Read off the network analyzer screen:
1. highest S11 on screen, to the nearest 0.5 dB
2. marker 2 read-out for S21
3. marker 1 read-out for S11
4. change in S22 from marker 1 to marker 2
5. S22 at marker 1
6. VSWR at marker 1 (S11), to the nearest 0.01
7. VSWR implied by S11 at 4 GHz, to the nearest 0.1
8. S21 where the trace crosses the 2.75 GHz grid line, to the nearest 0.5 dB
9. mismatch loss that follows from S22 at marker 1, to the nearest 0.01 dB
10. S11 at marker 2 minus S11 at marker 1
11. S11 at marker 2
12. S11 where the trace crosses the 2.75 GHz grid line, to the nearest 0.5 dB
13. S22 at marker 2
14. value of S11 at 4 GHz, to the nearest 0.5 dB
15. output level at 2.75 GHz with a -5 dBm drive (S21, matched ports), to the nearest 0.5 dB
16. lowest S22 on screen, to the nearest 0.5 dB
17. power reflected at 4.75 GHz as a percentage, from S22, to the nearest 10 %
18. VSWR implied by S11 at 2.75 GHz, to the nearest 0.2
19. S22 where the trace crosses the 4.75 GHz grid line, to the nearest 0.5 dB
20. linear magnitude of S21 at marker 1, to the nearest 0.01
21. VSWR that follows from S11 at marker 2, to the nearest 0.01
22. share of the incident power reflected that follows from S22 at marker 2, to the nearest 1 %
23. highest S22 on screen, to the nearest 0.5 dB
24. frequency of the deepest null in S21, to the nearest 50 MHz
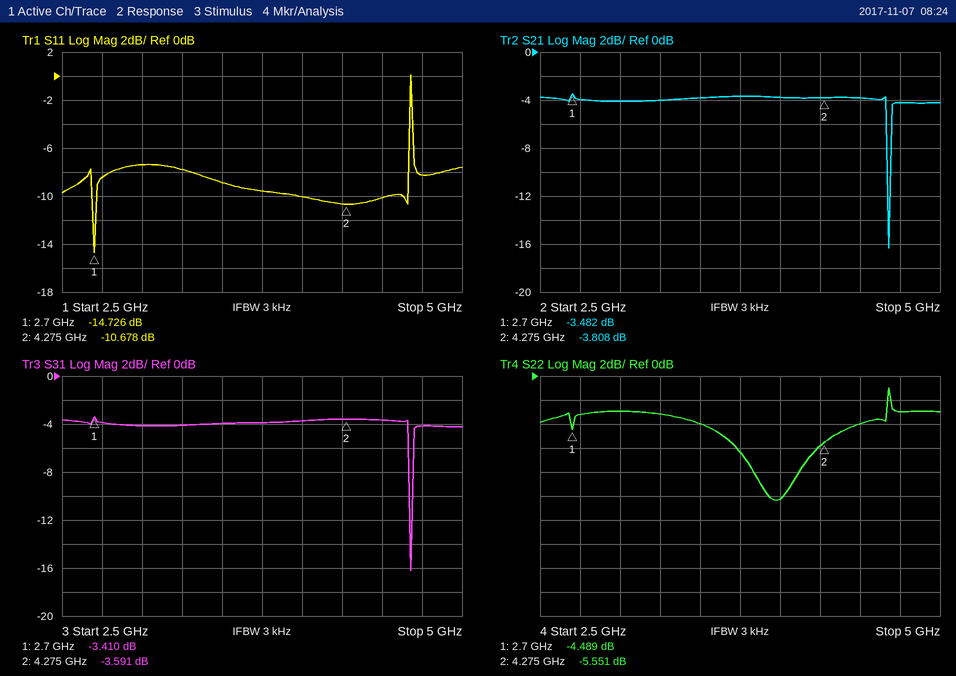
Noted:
0.0 dB
-3.808 dB
-14.726 dB
-1.062 dB
-4.489 dB
1.45
1.9
-4.0 dB
1.91 dB
4.048 dB
-10.678 dB
-8.5 dB
-5.551 dB
-10.0 dB
-9.0 dBm
-10.5 dB
50 %
2.2
-3.0 dB
0.67
1.83
28 %
-1.0 dB
4.70 GHz
